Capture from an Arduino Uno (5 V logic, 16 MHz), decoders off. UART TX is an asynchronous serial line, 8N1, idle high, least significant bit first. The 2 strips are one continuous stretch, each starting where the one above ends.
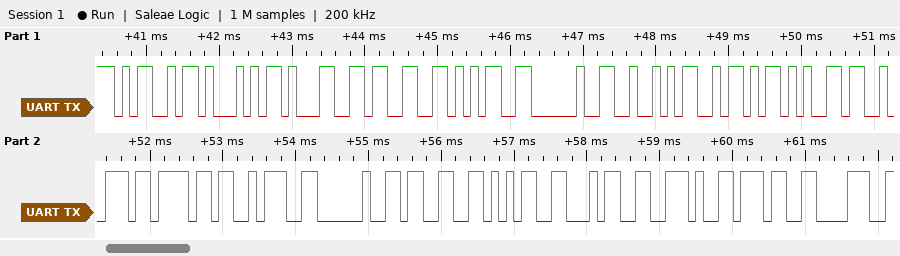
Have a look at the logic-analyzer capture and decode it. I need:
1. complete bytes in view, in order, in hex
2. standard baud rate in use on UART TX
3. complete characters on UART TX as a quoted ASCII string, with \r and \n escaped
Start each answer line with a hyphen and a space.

- 0x4D 0x51 0x31 0x33 0x35 0x20 0x52 0x5A 0x65 0x72 0x6F 0x3A 0x20 0x33 0x35 0x34 0x2E 0x37 0x38
- 9600 baud
- "MQ135 RZero: 354.78"
